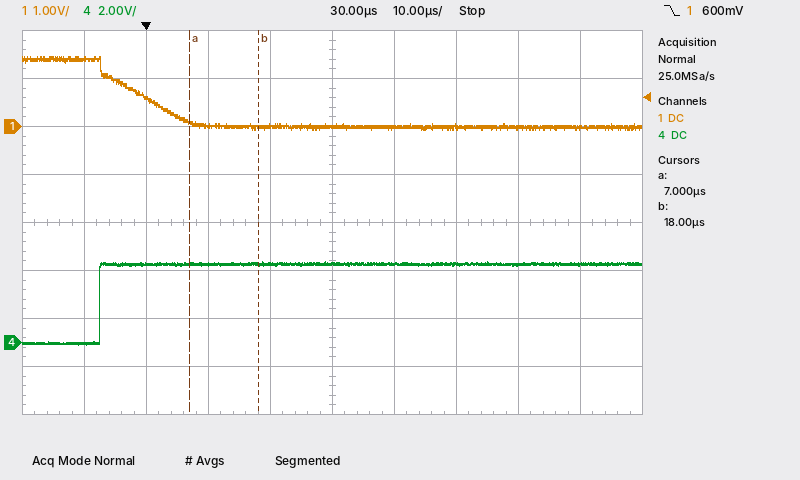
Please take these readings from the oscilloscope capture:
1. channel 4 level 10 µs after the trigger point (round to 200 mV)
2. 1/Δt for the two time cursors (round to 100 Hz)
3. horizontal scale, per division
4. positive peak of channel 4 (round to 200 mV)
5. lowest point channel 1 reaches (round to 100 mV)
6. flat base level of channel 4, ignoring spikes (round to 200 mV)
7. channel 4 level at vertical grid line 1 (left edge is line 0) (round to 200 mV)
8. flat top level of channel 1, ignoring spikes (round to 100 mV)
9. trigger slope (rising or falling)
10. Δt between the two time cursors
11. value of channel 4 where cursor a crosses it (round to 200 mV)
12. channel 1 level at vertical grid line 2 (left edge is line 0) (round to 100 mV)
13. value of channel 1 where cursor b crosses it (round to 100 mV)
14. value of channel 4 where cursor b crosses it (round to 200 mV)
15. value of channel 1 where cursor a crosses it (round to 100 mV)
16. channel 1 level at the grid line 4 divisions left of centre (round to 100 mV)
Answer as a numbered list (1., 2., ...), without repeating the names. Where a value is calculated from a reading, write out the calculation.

1. 3.2 V
2. 1 / 11 µs ≈ 90.9 kHz
3. 10 µs
4. 3.4 V
5. -100 mV
6. 0.0 V
7. 0.0 V
8. 1.4 V
9. falling
10. 18 µs − (7 µs) = 11 µs
11. 3.2 V
12. 600 mV
13. 0.0 V
14. 3.2 V
15. 100 mV
16. 1.4 V
